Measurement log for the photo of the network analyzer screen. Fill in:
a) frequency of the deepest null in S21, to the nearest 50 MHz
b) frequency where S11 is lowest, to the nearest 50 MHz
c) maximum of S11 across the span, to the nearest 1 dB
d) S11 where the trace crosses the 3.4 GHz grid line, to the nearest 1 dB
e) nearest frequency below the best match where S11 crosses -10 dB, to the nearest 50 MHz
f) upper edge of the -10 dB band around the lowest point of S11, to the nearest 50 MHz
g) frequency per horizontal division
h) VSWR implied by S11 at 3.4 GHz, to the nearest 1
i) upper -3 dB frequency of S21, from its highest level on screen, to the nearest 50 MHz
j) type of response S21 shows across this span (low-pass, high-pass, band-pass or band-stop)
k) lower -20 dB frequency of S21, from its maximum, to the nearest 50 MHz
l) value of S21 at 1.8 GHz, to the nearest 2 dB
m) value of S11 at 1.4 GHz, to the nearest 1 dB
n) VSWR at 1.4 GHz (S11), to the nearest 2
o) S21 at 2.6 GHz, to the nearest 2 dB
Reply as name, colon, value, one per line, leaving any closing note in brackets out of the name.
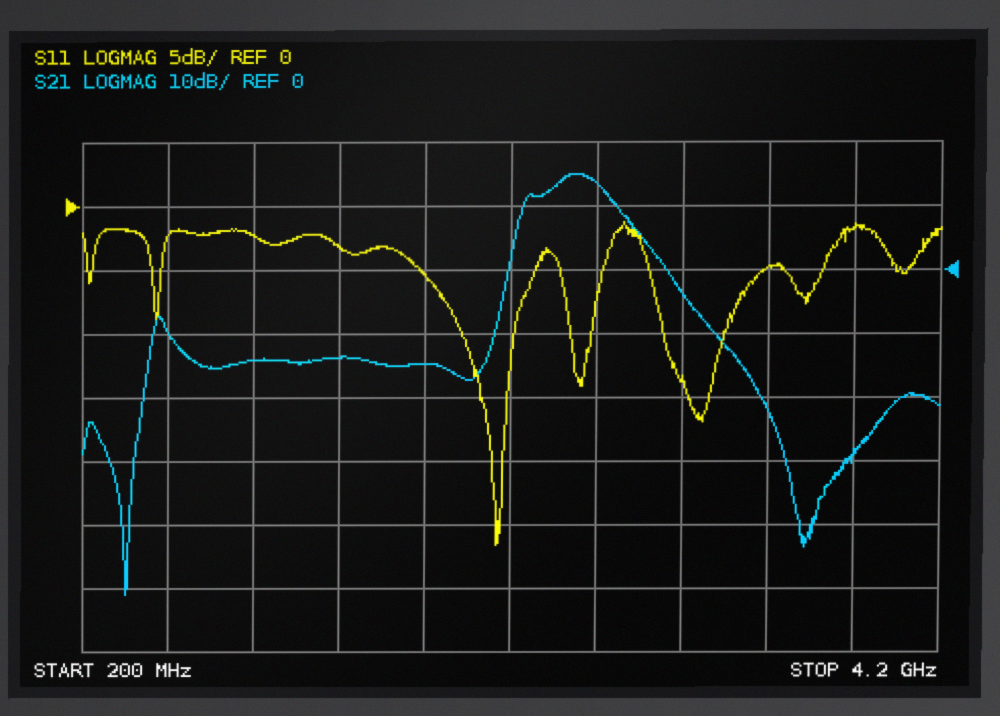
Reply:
frequency of the deepest null in S21, to the nearest 50 MHz: 400 MHz
frequency where S11 is lowest, to the nearest 50 MHz: 2.15 GHz
maximum of S11 across the span, to the nearest 1 dB: -1 dB
S11 where the trace crosses the 3.4 GHz grid line, to the nearest 1 dB: -5 dB
nearest frequency below the best match where S11 crosses -10 dB, to the nearest 50 MHz: 1.95 GHz
upper edge of the -10 dB band around the lowest point of S11, to the nearest 50 MHz: 2.20 GHz
frequency per horizontal division: 400 MHz
VSWR implied by S11 at 3.4 GHz, to the nearest 1: 4
upper -3 dB frequency of S21, from its highest level on screen, to the nearest 50 MHz: 2.65 GHz
type of response S21 shows across this span: band-pass
lower -20 dB frequency of S21, from its maximum, to the nearest 50 MHz: 2.15 GHz
value of S21 at 1.8 GHz, to the nearest 2 dB: -14 dB
value of S11 at 1.4 GHz, to the nearest 1 dB: -3 dB
VSWR at 1.4 GHz (S11), to the nearest 2: 6
S21 at 2.6 GHz, to the nearest 2 dB: 14 dB
